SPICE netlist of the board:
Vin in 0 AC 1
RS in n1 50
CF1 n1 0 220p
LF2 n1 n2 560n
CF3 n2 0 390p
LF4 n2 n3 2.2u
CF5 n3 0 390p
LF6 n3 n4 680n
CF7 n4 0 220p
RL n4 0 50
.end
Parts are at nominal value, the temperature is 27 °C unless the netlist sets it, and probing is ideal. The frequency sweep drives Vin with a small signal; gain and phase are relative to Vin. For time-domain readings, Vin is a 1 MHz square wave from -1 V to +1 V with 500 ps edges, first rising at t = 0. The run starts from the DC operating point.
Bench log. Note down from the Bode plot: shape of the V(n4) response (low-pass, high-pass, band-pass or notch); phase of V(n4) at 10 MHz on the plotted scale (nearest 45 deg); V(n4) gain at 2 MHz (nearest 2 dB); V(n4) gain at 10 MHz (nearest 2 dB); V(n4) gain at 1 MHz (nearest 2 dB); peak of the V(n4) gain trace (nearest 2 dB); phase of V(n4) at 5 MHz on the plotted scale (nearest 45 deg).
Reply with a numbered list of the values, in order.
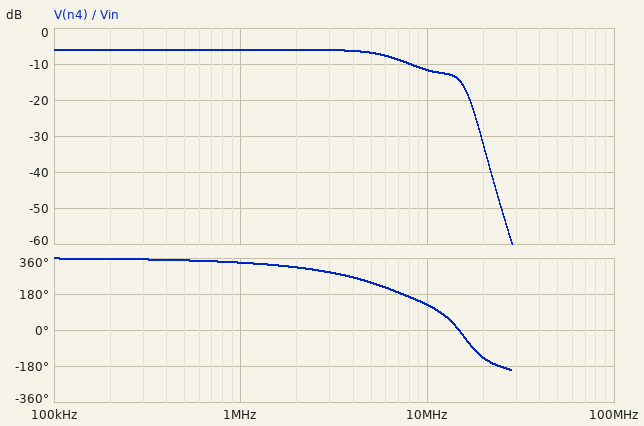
1. low-pass
2. 135 deg
3. -6 dB
4. -12 dB
5. -6 dB
6. -6 dB
7. 225 deg
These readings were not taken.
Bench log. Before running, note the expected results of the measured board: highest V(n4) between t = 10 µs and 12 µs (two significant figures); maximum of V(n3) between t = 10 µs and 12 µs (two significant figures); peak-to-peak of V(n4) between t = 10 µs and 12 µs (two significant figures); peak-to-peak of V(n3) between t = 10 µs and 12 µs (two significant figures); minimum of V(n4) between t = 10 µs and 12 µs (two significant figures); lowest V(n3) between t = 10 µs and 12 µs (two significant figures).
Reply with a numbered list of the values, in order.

1. 550 mV
2. 560 mV
3. 1.1 V
4. 1.1 V
5. -550 mV
6. -560 mV
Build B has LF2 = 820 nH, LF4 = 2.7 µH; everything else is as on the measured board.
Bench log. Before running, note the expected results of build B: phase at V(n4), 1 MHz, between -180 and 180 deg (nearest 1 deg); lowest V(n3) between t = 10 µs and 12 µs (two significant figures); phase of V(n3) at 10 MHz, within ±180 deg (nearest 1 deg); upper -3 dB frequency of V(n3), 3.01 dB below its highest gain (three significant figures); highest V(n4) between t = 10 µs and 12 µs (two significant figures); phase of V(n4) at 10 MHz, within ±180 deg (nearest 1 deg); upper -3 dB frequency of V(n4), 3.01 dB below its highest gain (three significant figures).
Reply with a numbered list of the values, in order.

1. -26 deg
2. -540 mV
3. 170 deg
4. 5.89 MHz
5. 540 mV
6. 105 deg
7. 6.41 MHz
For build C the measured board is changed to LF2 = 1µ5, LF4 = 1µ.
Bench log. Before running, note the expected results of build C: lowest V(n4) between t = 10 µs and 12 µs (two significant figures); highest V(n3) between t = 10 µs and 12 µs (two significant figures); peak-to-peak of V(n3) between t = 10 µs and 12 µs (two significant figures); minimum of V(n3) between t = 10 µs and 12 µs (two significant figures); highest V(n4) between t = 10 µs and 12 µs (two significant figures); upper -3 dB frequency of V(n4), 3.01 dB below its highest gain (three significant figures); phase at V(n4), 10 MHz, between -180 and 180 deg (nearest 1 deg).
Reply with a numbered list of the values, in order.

1. -630 mV
2. 580 mV
3. 1.2 V
4. -580 mV
5. 630 mV
6. 12.6 MHz
7. 120 deg
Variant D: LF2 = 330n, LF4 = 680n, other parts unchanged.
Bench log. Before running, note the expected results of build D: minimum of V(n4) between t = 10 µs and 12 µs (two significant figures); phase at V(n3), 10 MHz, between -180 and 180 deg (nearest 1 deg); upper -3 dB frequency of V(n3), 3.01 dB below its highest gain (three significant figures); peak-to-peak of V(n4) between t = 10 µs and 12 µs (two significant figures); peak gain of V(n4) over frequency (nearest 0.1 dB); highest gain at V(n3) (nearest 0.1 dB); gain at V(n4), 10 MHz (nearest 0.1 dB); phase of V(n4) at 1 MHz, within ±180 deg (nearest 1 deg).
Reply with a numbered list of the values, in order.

1. -630 mV
2. -108 deg
3. 19.2 MHz
4. 1.3 V
5. -6.0 dB
6. -3.6 dB
7. -6.5 dB
8. -17 deg
